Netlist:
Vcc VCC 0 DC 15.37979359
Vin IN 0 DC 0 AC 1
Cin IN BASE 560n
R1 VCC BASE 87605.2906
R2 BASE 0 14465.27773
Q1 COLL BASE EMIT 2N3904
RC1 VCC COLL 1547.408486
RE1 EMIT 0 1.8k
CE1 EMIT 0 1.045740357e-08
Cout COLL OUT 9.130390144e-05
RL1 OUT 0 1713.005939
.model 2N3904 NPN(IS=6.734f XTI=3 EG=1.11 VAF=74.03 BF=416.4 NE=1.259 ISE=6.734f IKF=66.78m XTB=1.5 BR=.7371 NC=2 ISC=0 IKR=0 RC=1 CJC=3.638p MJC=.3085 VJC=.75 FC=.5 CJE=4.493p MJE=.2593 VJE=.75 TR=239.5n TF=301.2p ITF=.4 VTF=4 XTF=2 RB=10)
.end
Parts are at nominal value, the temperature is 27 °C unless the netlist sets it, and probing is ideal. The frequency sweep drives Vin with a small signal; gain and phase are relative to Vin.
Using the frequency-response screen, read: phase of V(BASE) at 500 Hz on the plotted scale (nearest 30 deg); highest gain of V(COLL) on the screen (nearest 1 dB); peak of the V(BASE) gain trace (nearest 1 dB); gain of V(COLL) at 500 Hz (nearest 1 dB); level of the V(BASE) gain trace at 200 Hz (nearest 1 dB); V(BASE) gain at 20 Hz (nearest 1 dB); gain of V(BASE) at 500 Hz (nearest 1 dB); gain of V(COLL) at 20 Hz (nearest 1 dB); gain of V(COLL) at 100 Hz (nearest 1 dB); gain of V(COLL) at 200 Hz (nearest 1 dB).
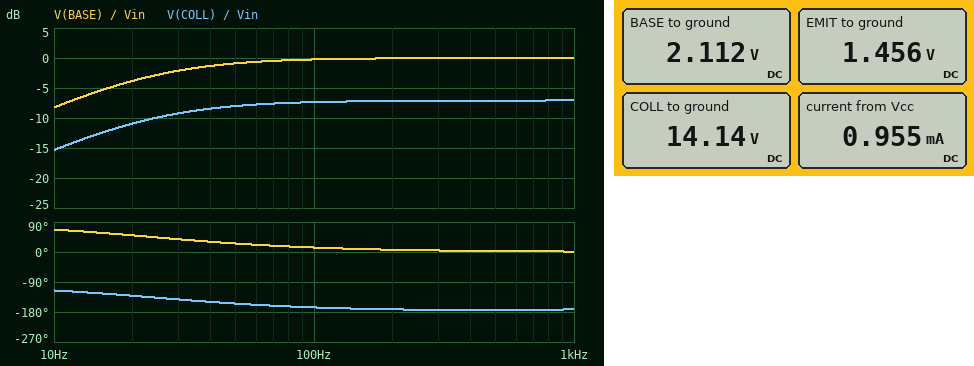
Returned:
0 deg
-7 dB
0 dB
-7 dB
0 dB
-4 dB
0 dB
-11 dB
-7 dB
-7 dB
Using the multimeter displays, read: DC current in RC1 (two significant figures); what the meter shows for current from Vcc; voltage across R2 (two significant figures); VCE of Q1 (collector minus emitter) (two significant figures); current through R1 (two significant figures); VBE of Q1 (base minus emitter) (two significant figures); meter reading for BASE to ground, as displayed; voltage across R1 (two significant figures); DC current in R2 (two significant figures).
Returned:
800 µA
0.955 mA
2.1 V
13 V
150 µA
660 mV
2.112 V
13 V
150 µA
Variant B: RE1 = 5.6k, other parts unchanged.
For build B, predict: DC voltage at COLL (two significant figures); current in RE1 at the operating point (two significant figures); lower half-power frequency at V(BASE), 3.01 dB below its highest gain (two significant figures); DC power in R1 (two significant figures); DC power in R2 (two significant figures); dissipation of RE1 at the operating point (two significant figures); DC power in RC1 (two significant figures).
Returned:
15 V
270 µA
23 Hz
2.0 mW
320 µW
420 µW
110 µW
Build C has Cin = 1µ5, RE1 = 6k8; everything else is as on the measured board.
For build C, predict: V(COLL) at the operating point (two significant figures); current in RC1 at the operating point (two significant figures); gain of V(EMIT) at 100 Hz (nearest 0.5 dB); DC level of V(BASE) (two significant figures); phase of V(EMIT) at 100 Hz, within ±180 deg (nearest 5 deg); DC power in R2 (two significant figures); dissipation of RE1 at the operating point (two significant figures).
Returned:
15 V
220 µA
0 dB
2.2 V
5 deg
320 µW
350 µW
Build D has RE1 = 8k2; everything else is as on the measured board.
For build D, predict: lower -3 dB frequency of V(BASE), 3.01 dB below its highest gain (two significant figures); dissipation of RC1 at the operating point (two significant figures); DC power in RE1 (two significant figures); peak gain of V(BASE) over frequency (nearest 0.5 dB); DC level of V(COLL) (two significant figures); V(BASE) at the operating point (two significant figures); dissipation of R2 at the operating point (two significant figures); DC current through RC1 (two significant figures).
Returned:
23 Hz
54 µW
290 µW
0 dB
15 V
2.2 V
320 µW
190 µA
